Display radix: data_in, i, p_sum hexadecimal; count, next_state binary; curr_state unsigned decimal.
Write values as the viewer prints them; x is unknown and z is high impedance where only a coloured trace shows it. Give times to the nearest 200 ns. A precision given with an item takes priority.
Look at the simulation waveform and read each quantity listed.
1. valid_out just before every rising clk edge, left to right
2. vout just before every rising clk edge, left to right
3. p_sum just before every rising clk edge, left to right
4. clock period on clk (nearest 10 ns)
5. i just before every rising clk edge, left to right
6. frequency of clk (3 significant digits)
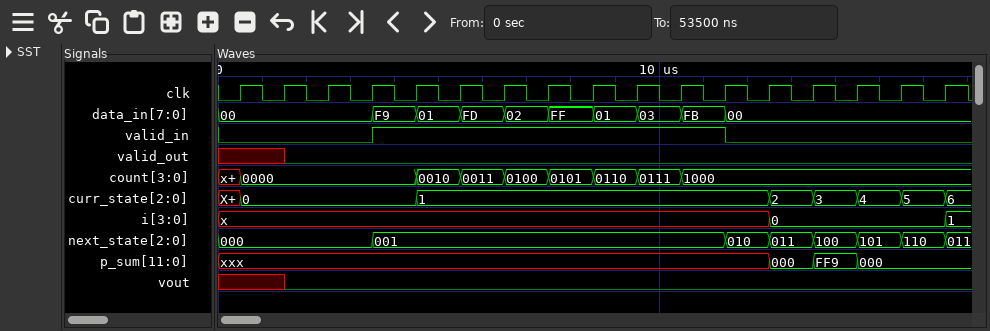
x x 0 0 0 0 0 0 0 0 0 0 0 0 0 0 0
x x 0 0 0 0 0 0 0 0 0 0 0 0 0 0 0
xxx, xxx, xxx, xxx, xxx, xxx, xxx, xxx, xxx, xxx, xxx, xxx, xxx, 000, FF9, 000, 000
1000 ns
x, x, x, x, x, x, x, x, x, x, x, x, x, 0, 0, 0, 0
1.00 MHz
